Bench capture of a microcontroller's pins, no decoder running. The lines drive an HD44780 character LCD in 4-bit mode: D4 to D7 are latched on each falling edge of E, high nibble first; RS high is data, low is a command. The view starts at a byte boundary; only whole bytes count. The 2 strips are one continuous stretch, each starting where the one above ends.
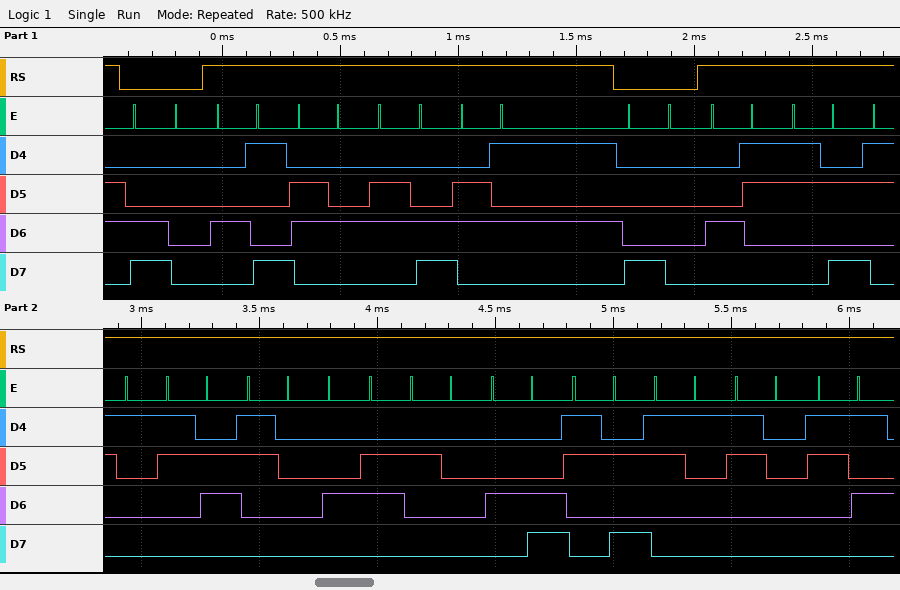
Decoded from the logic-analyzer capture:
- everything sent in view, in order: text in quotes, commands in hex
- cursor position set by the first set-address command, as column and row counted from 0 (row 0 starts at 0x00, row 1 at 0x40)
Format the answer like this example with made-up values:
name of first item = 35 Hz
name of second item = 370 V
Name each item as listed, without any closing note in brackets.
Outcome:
everything sent in view, in order: text in quotes, commands in hex = 0xC0 "Idle" 0x80 "C:160F L:105"
cursor position set by the first set-address command, as column and row counted from 0 = column 0, row 1
